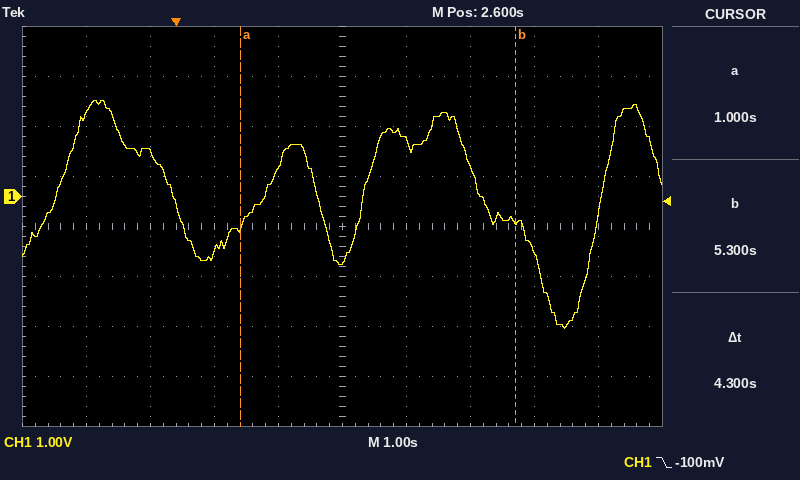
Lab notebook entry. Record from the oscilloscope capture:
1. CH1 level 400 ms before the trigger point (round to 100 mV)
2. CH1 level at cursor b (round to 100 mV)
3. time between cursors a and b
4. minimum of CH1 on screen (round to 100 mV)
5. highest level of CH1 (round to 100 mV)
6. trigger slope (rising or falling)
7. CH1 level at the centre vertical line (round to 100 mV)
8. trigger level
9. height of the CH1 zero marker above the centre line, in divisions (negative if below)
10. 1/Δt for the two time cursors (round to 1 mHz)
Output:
900 mV
-500 mV
4.3 s
-2.6 V
1.9 V
falling
-1.3 V
-100 mV
+0.6 div
233 mHz
